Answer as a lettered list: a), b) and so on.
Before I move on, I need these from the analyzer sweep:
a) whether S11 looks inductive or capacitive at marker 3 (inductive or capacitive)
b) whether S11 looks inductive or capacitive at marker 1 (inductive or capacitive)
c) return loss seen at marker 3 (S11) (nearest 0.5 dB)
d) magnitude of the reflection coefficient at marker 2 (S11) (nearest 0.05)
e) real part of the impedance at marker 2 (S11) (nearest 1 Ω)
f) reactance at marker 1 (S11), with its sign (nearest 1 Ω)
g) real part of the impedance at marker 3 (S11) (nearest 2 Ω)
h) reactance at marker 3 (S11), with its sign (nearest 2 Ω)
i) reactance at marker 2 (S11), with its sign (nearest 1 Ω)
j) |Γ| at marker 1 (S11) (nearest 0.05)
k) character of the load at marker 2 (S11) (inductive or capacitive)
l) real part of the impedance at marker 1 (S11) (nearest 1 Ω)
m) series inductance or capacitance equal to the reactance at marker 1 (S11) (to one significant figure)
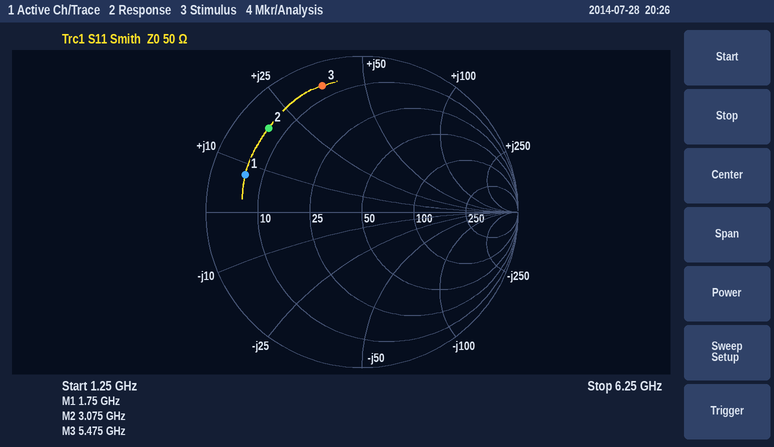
a) inductive
b) inductive
c) 1.5 dB
d) 0.80
e) 6 Ω
f) +8 Ω
g) 6 Ω
h) +36 Ω
i) +19 Ω
j) 0.80
k) inductive
l) 6 Ω
m) 700 pH
